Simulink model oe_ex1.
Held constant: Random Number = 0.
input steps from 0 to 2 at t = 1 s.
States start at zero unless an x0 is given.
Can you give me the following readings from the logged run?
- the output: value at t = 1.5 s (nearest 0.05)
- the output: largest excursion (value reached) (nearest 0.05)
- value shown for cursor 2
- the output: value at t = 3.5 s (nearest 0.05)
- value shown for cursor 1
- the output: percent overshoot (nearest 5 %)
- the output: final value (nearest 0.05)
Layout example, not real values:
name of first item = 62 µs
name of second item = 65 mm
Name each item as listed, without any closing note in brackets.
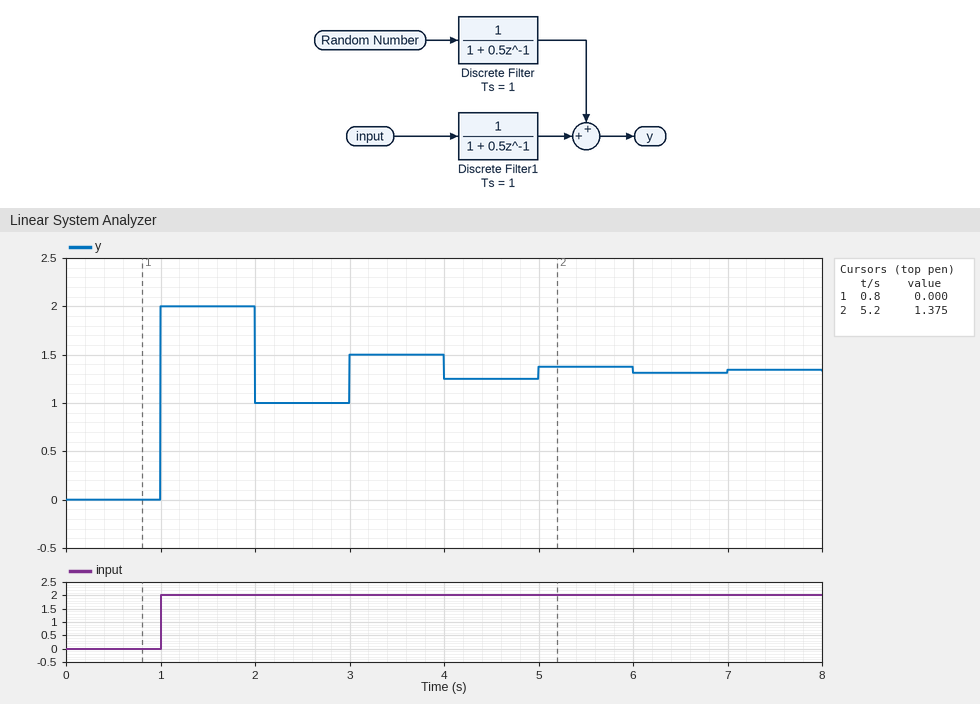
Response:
the output: value at t = 1.5 s = 2.00
the output: largest excursion (value reached) = 2.00
value shown for cursor 2 = 1.375
the output: value at t = 3.5 s = 1.50
value shown for cursor 1 = 0.000
the output: percent overshoot = 50 %
the output: final value = 1.35
